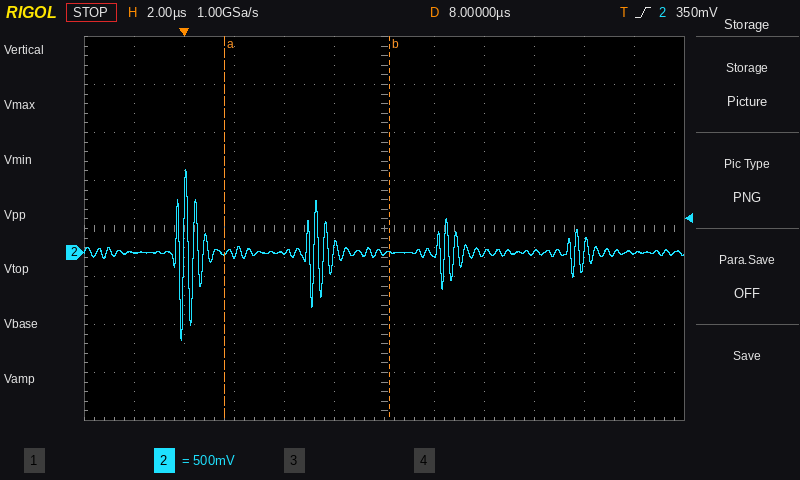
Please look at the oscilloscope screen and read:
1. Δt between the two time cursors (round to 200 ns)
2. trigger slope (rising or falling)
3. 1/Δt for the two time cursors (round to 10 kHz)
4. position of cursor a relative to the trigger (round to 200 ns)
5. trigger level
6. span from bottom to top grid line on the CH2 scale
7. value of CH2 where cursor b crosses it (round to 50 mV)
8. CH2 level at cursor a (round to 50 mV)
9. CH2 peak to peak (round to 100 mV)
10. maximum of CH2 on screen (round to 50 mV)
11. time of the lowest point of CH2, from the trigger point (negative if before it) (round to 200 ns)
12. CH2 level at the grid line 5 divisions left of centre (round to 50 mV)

6.6 µs
rising
150 kHz
+1.6 µs
350 mV
4 V
0 mV
0 mV
1.80 V
850 mV
-200 ns
0 mV
